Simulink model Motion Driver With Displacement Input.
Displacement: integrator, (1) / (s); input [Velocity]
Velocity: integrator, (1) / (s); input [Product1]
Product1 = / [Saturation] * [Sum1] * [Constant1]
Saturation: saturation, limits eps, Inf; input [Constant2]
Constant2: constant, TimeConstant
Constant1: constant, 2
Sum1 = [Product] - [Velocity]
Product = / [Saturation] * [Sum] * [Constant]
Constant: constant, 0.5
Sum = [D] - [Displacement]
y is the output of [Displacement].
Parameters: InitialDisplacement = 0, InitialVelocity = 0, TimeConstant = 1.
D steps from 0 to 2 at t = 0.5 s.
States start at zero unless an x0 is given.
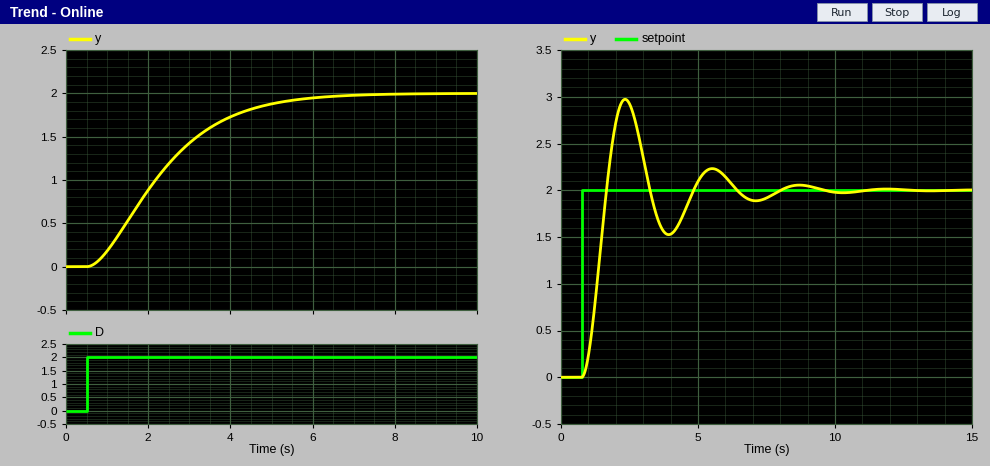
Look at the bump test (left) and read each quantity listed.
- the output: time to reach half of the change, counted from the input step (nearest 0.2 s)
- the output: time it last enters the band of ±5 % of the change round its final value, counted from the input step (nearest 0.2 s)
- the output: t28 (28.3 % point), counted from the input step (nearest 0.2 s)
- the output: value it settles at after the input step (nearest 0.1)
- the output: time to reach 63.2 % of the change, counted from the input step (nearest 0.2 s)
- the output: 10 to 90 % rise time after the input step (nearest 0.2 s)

1.6 s
4.8 s
1.0 s
2.0
2.2 s
3.4 s
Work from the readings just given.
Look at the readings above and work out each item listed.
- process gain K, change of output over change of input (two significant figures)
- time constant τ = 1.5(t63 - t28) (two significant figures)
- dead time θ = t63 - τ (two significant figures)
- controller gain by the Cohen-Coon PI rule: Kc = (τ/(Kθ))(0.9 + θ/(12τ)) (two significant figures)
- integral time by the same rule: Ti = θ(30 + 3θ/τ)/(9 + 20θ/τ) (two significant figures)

1.0
1.8 s
0.40 s
4.1
0.91 s
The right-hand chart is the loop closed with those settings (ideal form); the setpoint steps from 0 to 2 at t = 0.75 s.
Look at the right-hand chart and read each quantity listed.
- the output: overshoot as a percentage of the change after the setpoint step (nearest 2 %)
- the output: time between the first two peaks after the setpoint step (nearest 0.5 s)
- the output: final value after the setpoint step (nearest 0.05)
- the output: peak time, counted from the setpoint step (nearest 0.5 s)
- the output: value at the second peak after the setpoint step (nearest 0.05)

48 %
3.0 s
2.00
1.5 s
2.25
